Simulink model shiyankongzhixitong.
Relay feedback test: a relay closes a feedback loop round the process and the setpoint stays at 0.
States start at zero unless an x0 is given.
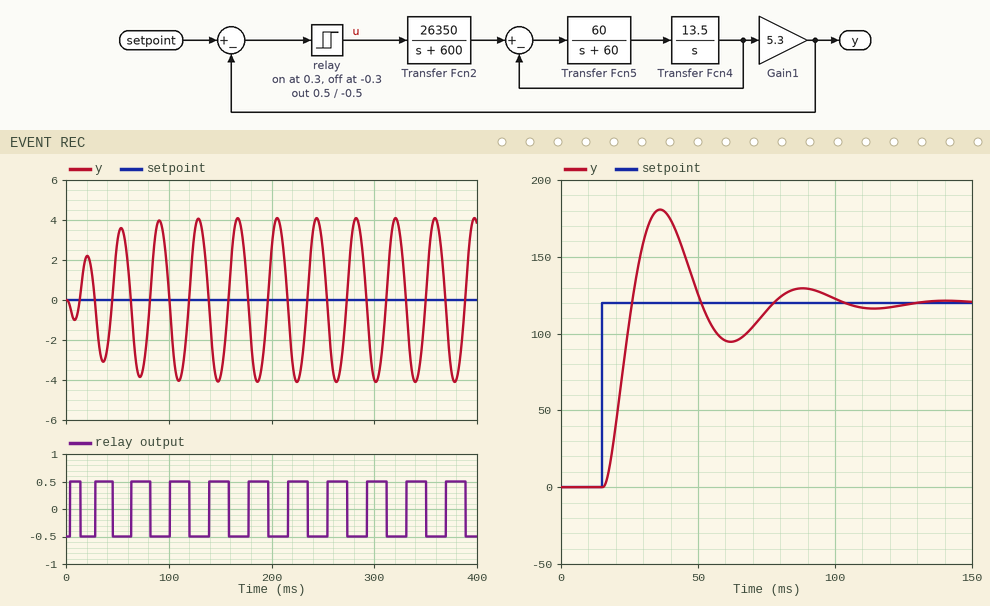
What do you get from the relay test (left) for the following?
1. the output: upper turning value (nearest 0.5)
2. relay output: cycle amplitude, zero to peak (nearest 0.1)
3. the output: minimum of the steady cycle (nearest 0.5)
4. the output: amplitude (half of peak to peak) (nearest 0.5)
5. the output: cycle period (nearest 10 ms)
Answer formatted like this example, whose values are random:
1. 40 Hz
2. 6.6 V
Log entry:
1. 4.0
2. 0.5
3. -4.0
4. 4.0
5. 40 ms
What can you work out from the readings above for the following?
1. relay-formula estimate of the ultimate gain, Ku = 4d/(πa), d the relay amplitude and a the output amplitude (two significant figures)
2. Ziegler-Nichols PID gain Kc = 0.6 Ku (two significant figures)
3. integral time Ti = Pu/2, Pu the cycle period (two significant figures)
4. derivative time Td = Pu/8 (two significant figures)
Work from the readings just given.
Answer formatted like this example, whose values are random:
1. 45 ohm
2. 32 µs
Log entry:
1. 0.16
2. 0.096
3. 20 ms
4. 5.0 ms
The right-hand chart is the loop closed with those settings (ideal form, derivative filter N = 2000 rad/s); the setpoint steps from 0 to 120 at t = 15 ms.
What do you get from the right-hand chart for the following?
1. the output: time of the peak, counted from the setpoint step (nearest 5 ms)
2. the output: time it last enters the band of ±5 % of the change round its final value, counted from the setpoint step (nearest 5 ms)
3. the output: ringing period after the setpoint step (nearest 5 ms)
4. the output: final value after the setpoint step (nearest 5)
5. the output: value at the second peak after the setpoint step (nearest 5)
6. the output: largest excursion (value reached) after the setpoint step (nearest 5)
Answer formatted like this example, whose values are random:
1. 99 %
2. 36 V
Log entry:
1. 20 ms
2. 80 ms
3. 50 ms
4. 120
5. 130
6. 180
